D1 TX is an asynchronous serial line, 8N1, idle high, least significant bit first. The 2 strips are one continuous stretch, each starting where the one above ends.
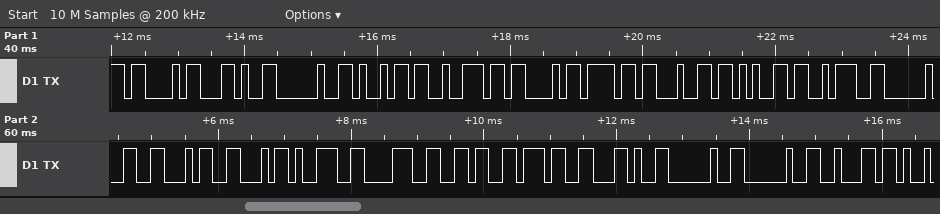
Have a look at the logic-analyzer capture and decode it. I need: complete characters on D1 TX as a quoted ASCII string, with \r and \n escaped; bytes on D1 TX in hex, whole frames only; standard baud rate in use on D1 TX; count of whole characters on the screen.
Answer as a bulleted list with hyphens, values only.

- "C, irCode: FF9867,  b"
- 0x43 0x2C 0x20 0x69 0x72 0x43 0x6F 0x64 0x65 0x3A 0x20 0x46 0x46 0x39 0x38 0x36 0x37 0x2C 0x20 0x20 0x62
- 9600 baud
- 21
